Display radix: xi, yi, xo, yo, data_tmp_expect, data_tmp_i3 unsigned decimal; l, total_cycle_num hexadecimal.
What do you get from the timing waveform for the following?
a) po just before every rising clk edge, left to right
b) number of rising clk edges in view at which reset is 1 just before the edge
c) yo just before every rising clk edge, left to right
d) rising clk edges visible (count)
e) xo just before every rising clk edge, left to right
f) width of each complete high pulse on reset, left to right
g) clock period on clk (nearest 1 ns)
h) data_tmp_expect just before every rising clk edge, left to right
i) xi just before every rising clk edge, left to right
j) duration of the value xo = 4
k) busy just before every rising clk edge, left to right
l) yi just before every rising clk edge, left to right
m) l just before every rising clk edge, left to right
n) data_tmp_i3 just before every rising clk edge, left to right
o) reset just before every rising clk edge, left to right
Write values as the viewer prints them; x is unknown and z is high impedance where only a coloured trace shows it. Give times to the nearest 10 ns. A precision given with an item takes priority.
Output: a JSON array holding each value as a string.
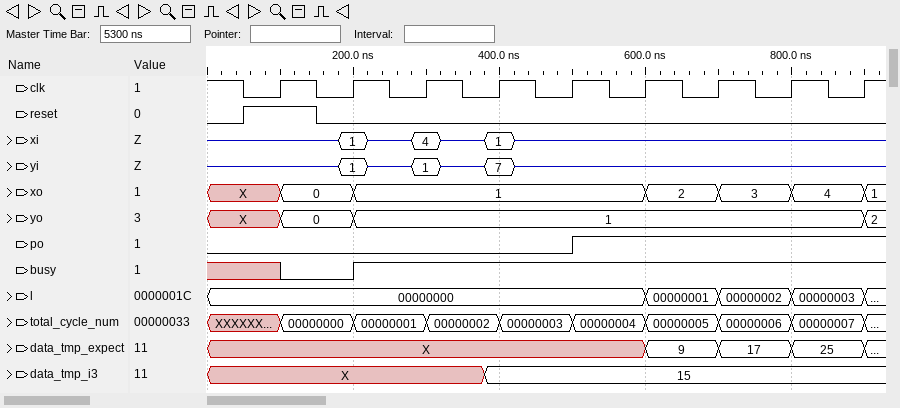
["0 0 0 0 0 1 1 1 1", "1", "X, 0, 1, 1, 1, 1, 1, 1, 1", "9", "X, 0, 1, 1, 1, 1, 2, 3, 4", "100 ns", "100 ns", "X, X, X, X, X, X, 9, 17, 25", "z, 1, 4, 1, z, z, z, z, z", "100 ns", "x 0 1 1 1 1 1 1 1", "z, 1, 1, 7, z, z, z, z, z", "00000000, 00000000, 00000000, 00000000, 00000000, 00000000, 00000001, 00000002, 00000003", "X, X, X, 15, 15, 15, 15, 15, 15", "1 0 0 0 0 0 0 0 0"]
